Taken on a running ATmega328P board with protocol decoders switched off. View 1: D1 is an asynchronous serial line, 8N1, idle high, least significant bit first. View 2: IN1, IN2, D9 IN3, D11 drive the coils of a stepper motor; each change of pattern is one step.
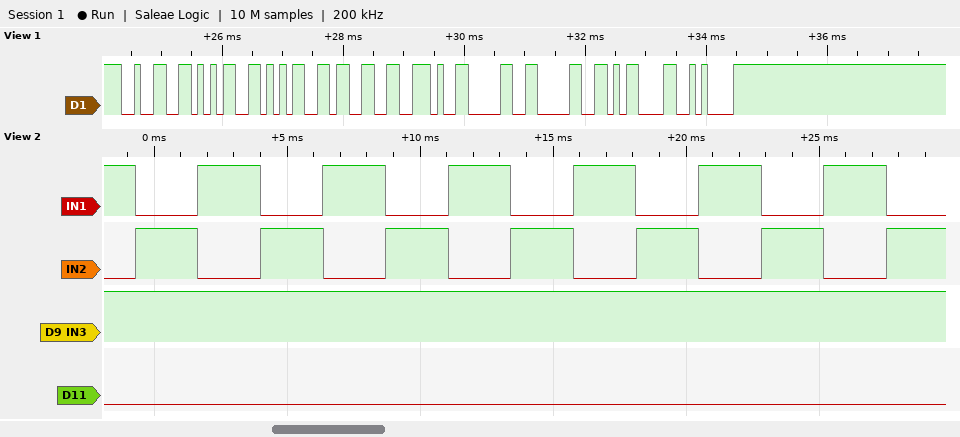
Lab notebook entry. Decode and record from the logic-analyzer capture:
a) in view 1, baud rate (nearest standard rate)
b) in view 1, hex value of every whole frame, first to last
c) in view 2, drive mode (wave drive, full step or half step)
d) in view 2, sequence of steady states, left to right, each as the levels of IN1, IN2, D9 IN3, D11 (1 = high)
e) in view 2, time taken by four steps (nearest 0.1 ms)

9600 baud
32 35 35 33 2E 30 30 0D 0A
full step
1010 0110 1010 0110 1010 0110 1010 0110 1010 0110 1010 0110 1010 0110
9.4 ms
